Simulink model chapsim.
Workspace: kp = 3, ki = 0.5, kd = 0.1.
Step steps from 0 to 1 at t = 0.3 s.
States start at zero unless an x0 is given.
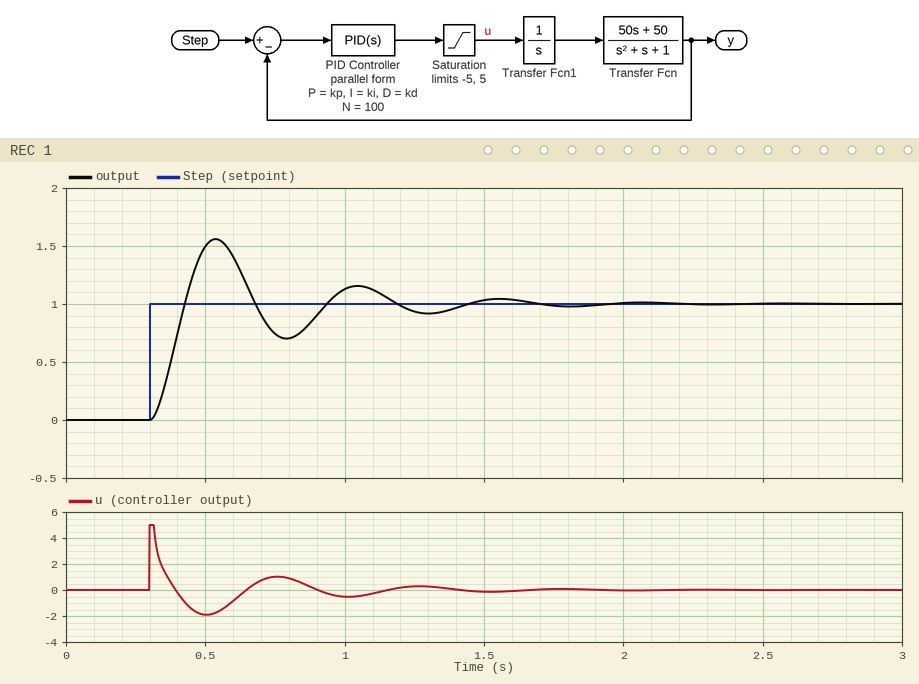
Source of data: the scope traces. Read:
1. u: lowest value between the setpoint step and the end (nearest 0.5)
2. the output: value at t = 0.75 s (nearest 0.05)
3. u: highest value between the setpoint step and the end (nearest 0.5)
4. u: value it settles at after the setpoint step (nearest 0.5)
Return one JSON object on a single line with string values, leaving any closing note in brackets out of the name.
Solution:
{"u: lowest value between the setpoint step and the end": "-2.0", "the output: value at t = 0.75 s": "0.75", "u: highest value between the setpoint step and the end": "5.0", "u: value it settles at after the setpoint step": "0.0"}
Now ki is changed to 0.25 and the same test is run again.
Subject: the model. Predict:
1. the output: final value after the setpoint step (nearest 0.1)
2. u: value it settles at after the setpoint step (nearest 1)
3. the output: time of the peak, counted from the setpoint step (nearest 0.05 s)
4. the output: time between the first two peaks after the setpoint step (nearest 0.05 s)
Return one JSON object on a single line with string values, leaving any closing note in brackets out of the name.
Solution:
{"the output: final value after the setpoint step": "1.0", "u: value it settles at after the setpoint step": "0", "the output: time of the peak, counted from the setpoint step": "0.25 s", "the output: time between the first two peaks after the setpoint step": "0.50 s"}
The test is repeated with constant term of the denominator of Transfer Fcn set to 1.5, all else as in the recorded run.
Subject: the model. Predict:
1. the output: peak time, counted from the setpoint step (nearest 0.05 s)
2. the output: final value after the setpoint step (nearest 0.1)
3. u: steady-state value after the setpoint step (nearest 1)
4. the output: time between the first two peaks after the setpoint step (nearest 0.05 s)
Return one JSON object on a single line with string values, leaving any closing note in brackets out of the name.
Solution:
{"the output: peak time, counted from the setpoint step": "0.25 s", "the output: final value after the setpoint step": "1.0", "u: steady-state value after the setpoint step": "0", "the output: time between the first two peaks after the setpoint step": "0.50 s"}
